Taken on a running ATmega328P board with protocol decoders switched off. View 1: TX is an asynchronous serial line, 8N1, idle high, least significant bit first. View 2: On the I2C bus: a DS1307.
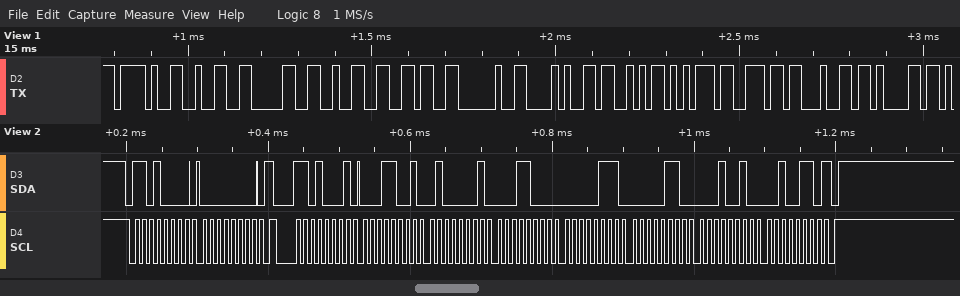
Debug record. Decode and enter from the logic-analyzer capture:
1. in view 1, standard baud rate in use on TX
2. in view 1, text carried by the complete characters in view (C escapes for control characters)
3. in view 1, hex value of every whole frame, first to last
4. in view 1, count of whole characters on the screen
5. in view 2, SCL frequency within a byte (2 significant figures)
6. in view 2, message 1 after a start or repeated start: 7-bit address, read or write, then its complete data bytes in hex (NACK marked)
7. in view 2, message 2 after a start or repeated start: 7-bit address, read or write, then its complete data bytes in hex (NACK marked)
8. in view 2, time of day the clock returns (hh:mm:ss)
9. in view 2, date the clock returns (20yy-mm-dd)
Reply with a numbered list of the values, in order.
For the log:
1. 57600 baud
2. "/2026 (Sunda"
3. 0x2F 0x32 0x30 0x32 0x36 0x20 0x28 0x53 0x75 0x6E 0x64 0x61
4. 12
5. 100 kHz
6. 0x68 write: 00
7. 0x68 read: 19 41 18 07 06 12 26 NACK
8. 18:41:19
9. 2026-12-06
